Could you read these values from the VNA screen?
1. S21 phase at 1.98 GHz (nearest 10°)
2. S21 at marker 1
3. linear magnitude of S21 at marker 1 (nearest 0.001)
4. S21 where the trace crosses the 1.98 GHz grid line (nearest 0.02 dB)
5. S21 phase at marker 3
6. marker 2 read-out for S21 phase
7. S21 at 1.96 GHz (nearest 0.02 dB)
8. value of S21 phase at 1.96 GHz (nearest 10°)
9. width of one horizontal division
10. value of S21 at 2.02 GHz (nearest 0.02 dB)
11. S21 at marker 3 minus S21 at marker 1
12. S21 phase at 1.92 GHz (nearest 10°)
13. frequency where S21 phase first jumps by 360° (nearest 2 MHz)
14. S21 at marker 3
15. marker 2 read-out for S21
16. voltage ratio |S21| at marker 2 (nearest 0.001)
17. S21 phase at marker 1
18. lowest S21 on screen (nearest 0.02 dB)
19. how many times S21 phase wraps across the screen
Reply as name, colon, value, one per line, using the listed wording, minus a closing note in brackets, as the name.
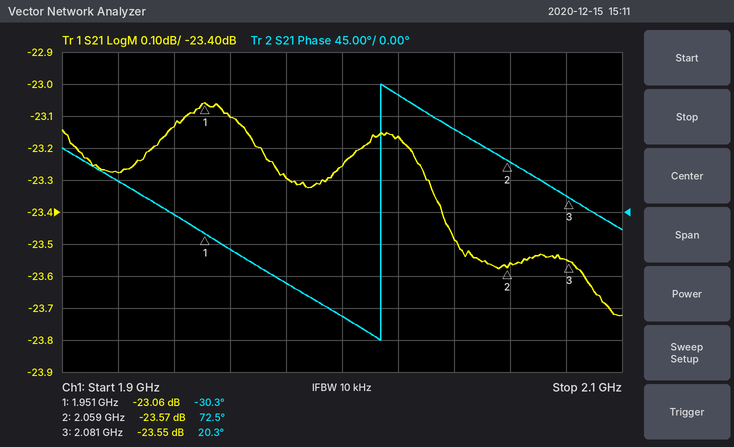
S21 phase at 1.98 GHz: -100°
S21 at marker 1: -23.06 dB
linear magnitude of S21 at marker 1: 0.070
S21 where the trace crosses the 1.98 GHz grid line: -23.30 dB
S21 phase at marker 3: 20.3°
marker 2 read-out for S21 phase: 72.5°
S21 at 1.96 GHz: -23.10 dB
value of S21 phase at 1.96 GHz: -50°
width of one horizontal division: 20 MHz
value of S21 at 2.02 GHz: -23.16 dB
S21 at marker 3 minus S21 at marker 1: -0.49 dB
S21 phase at 1.92 GHz: 40°
frequency where S21 phase first jumps by 360°: 2.014 GHz
S21 at marker 3: -23.55 dB
marker 2 read-out for S21: -23.57 dB
voltage ratio |S21| at marker 2: 0.066
S21 phase at marker 1: -30.3°
lowest S21 on screen: -23.72 dB
how many times S21 phase wraps across the screen: 1
